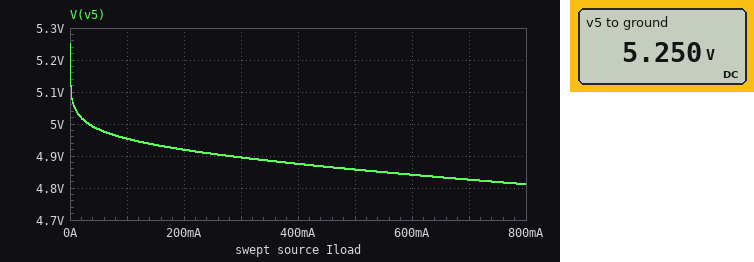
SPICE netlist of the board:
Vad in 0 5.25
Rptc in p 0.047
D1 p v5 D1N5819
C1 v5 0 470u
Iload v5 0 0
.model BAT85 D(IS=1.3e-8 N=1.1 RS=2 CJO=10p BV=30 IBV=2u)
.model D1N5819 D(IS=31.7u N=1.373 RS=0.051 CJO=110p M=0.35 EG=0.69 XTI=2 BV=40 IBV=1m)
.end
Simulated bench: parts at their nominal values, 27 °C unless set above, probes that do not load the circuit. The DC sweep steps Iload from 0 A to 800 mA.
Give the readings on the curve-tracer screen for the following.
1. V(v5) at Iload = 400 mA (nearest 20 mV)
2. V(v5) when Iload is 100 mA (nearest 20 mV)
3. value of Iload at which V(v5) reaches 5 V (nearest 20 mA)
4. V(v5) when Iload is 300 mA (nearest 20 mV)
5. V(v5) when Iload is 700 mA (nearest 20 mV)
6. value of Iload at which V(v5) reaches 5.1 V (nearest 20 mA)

4.88 V
4.96 V
40 mA
4.90 V
4.82 V
0 A
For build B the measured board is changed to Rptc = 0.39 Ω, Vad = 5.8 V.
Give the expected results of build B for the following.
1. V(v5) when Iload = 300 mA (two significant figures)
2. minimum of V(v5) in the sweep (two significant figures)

5.3 V
5.1 V
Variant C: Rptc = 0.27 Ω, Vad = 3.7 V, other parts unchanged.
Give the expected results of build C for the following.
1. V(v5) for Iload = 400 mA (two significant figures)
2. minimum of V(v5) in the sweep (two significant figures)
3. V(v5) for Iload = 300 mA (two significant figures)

3.2 V
3.1 V
3.3 V
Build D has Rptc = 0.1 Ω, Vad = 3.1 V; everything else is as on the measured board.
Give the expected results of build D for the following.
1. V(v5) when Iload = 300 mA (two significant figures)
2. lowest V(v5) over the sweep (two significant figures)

2.7 V
2.6 V
